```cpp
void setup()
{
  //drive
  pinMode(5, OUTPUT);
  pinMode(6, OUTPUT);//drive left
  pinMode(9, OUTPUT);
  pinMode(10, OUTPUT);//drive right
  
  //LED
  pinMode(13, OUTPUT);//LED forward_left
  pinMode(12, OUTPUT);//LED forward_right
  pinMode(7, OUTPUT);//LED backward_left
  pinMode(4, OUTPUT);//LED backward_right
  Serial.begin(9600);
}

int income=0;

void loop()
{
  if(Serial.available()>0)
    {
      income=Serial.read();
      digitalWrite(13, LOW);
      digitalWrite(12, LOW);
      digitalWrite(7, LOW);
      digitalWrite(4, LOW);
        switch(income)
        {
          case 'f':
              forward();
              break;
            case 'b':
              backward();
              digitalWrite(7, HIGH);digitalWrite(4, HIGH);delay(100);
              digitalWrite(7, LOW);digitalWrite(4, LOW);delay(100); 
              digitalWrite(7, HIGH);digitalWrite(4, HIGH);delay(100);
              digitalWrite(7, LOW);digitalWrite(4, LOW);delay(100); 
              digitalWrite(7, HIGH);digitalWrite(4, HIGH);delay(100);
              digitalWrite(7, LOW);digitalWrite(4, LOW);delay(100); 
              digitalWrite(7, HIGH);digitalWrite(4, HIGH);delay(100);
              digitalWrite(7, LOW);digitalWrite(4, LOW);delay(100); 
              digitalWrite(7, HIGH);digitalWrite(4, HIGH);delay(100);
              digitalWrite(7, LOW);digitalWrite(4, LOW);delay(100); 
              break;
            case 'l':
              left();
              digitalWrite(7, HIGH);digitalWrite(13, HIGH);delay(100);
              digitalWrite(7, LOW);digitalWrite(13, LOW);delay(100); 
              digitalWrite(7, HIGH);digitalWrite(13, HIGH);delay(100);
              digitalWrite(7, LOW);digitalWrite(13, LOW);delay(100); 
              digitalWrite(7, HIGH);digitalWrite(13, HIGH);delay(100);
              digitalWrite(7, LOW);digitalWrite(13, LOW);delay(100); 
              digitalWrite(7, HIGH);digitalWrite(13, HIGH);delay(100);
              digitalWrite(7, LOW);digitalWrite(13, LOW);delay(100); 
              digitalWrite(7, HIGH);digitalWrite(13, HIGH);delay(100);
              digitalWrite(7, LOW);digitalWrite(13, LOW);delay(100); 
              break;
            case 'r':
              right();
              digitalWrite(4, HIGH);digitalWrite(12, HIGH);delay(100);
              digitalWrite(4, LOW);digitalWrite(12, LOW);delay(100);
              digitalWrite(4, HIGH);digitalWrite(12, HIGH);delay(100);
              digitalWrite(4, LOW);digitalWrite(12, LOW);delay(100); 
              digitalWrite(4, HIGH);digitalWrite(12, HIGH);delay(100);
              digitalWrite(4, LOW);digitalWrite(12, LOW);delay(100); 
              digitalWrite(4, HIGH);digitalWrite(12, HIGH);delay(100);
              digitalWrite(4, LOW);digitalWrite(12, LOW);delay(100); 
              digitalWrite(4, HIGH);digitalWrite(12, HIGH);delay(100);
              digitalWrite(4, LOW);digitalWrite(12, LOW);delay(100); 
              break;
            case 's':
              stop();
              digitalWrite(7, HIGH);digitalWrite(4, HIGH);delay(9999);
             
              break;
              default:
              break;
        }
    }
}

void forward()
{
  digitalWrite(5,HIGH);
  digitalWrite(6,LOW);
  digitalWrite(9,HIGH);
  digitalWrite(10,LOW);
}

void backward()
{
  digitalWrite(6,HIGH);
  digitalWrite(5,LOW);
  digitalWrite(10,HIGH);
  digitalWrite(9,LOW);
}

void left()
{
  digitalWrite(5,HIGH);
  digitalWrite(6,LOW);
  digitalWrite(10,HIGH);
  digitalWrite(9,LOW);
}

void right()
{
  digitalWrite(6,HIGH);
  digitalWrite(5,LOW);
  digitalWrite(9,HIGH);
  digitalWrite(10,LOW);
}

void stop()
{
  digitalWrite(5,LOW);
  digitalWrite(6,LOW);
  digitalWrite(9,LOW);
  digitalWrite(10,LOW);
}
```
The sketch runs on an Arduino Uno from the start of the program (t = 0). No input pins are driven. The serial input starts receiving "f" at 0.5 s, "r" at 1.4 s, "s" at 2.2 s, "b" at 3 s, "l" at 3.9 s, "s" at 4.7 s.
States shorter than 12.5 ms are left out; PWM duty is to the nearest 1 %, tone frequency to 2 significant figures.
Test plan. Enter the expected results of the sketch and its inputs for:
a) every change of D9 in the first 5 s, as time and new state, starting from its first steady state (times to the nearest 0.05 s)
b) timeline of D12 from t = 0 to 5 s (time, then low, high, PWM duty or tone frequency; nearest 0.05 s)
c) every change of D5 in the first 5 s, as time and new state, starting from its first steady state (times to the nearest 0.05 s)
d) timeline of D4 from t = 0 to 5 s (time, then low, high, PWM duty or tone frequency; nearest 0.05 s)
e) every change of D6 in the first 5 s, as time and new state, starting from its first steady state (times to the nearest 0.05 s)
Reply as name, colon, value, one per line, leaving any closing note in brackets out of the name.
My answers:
every change of D9 in the first 5 s, as time and new state, starting from its first steady state: 0 s low; 0.5 s high; 2.4 s low
timeline of D12 from t = 0 to 5 s: 0 s low; 1.4 s high; 1.5 s low; 1.6 s high; 1.7 s low; 1.8 s high; 1.9 s low; 2 s high; 2.1 s low; 2.2 s high; 2.3 s low
every change of D5 in the first 5 s, as time and new state, starting from its first steady state: 0 s low; 0.5 s high; 1.4 s low
timeline of D4 from t = 0 to 5 s: 0 s low; 1.4 s high; 1.5 s low; 1.6 s high; 1.7 s low; 1.8 s high; 1.9 s low; 2 s high; 2.1 s low; 2.2 s high; 2.3 s low; 2.4 s high
every change of D6 in the first 5 s, as time and new state, starting from its first steady state: 0 s low; 1.4 s high; 2.4 s low
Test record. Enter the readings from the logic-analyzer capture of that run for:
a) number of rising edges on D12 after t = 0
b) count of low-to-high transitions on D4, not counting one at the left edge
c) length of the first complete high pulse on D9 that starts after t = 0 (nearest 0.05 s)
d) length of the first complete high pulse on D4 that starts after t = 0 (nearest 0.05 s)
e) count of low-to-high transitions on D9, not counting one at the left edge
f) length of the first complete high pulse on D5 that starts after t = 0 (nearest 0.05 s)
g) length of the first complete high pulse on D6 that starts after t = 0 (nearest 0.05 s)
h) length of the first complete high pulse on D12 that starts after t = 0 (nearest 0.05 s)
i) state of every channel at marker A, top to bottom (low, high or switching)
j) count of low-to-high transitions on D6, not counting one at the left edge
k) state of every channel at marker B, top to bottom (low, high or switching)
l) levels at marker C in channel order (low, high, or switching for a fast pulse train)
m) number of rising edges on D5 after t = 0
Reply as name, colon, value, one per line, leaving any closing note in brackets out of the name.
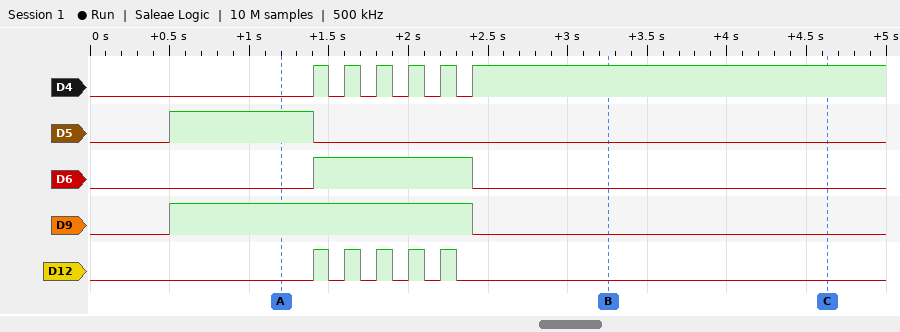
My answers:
number of rising edges on D12 after t = 0: 5
count of low-to-high transitions on D4, not counting one at the left edge: 6
length of the first complete high pulse on D9 that starts after t = 0: 1.90 s
length of the first complete high pulse on D4 that starts after t = 0: 0.10 s
count of low-to-high transitions on D9, not counting one at the left edge: 1
length of the first complete high pulse on D5 that starts after t = 0: 0.90 s
length of the first complete high pulse on D6 that starts after t = 0: 1.00 s
length of the first complete high pulse on D12 that starts after t = 0: 0.10 s
state of every channel at marker A, top to bottom: D4 low, D5 high, D6 low, D9 high, D12 low
count of low-to-high transitions on D6, not counting one at the left edge: 1
state of every channel at marker B, top to bottom: D4 high, D5 low, D6 low, D9 low, D12 low
levels at marker C in channel order: D4 high, D5 low, D6 low, D9 low, D12 low
number of rising edges on D5 after t = 0: 1
